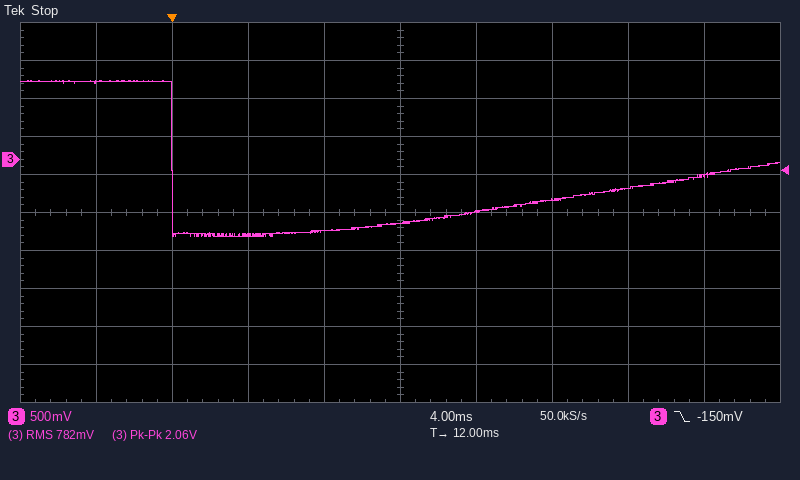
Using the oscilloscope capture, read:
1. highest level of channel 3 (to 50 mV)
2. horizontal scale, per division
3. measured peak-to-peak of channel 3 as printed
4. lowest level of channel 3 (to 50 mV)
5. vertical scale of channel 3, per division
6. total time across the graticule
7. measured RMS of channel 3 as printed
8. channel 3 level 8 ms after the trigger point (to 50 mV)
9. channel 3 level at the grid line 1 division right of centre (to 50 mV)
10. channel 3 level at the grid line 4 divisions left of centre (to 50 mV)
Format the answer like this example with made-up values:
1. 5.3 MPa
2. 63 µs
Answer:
1. 1.05 V
2. 4 ms
3. 2.06 V
4. -1.00 V
5. 500 mV
6. 40 ms
7. 782 mV
8. -950 mV
9. -700 mV
10. 1.00 V
